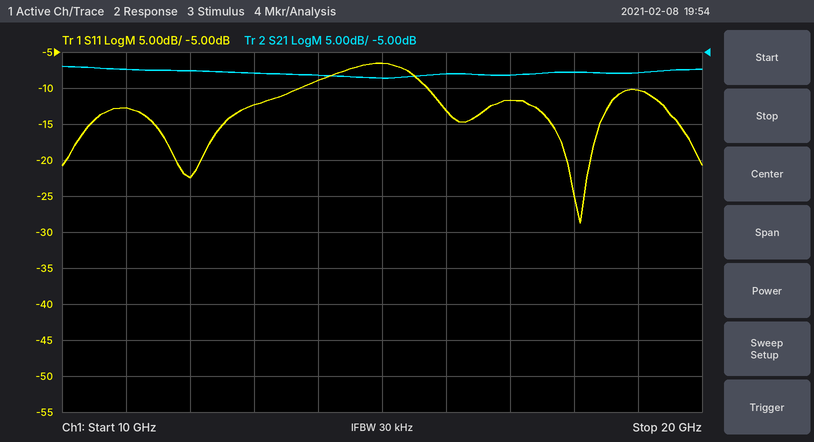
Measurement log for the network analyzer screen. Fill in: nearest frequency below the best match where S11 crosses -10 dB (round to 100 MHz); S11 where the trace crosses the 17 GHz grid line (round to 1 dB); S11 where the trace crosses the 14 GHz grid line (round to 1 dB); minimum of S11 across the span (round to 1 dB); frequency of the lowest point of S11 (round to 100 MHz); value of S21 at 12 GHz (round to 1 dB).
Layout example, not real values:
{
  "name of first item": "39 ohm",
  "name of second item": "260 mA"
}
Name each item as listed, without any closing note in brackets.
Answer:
{
  "nearest frequency below the best match where S11 crosses -10 dB": "15.7 GHz",
  "S11 where the trace crosses the 17 GHz grid line": "-12 dB",
  "S11 where the trace crosses the 14 GHz grid line": "-9 dB",
  "minimum of S11 across the span": "-29 dB",
  "frequency of the lowest point of S11": "18.1 GHz",
  "value of S21 at 12 GHz": "-8 dB"
}
